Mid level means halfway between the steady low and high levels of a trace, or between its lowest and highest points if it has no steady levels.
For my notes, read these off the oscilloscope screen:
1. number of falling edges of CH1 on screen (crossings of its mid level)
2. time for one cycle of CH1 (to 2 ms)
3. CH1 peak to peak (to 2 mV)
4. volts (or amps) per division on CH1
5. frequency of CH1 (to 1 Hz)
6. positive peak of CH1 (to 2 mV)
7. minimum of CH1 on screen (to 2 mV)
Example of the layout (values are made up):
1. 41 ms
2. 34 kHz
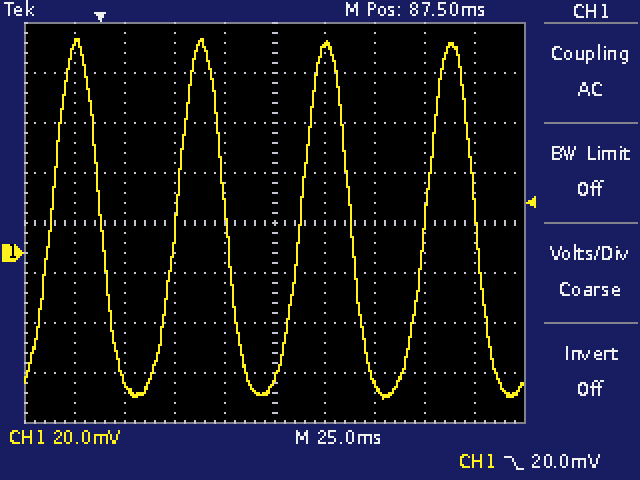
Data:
1. 4
2. 62 ms
3. 144 mV
4. 20 mV
5. 16 Hz
6. 86 mV
7. -58 mV
